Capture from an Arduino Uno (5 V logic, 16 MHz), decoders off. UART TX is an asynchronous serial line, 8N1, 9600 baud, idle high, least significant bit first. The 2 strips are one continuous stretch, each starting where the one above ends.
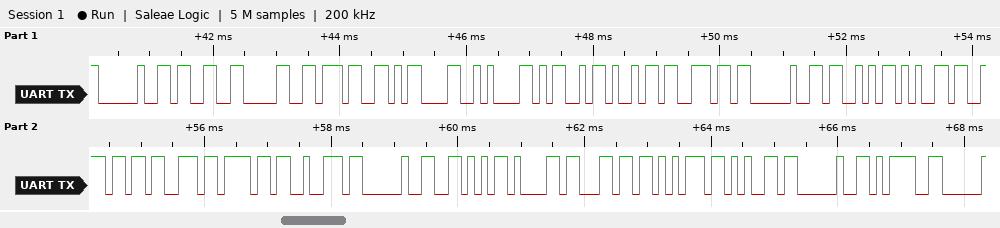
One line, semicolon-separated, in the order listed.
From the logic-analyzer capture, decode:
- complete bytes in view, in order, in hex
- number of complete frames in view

0x20 0x33 0x30 0x37 0x0D 0x0A 0x4D 0x69 0x6E 0x20 0x53 0x65 0x6E 0x73 0x6F 0x72 0x20 0x56 0x61 0x6C 0x75 0x65 0x20 0x3D; 24
